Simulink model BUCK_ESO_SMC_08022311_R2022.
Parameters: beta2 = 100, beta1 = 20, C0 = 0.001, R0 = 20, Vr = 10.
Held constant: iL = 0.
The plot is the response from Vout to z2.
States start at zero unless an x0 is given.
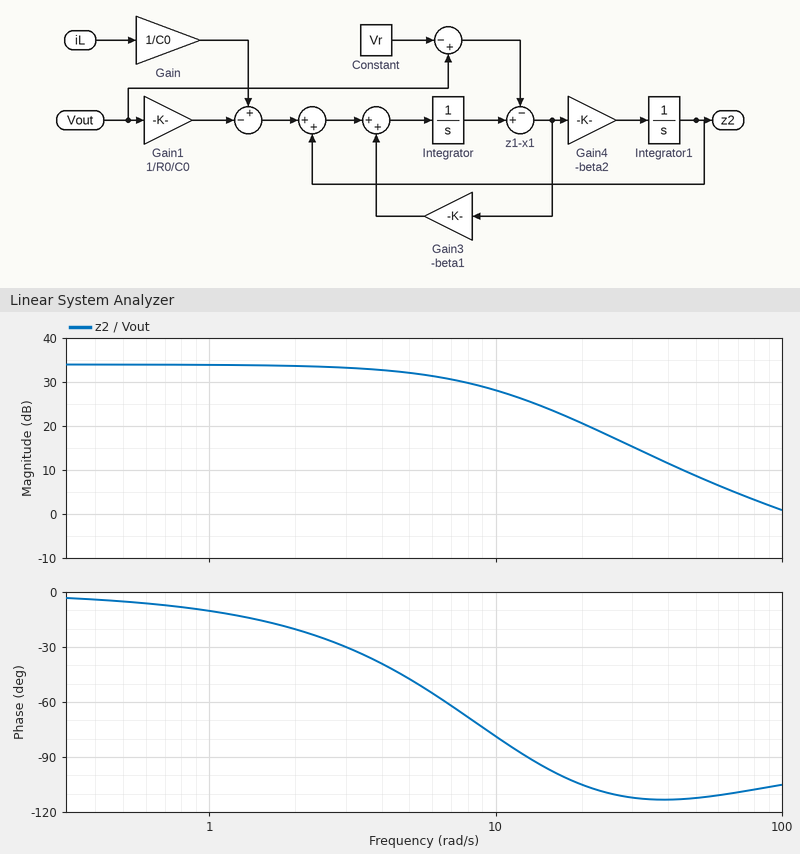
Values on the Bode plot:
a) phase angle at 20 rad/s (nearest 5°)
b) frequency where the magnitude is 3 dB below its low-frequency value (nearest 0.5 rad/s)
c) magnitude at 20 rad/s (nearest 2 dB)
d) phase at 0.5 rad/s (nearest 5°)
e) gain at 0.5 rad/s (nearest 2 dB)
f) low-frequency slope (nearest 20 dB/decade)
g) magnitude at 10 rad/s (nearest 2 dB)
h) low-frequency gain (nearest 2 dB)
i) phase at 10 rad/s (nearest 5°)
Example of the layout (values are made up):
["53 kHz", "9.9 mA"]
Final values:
["-105°", "6.5 rad/s", "20 dB", "-5°", "34 dB", "0 dB/decade", "28 dB", "34 dB", "-80°"]
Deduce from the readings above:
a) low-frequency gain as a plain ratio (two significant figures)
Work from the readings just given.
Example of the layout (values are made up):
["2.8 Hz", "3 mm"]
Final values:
["50"]
